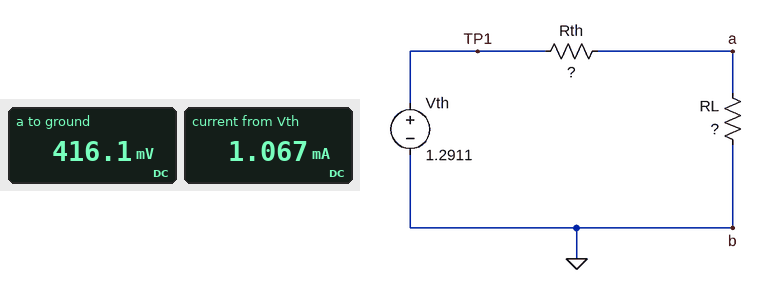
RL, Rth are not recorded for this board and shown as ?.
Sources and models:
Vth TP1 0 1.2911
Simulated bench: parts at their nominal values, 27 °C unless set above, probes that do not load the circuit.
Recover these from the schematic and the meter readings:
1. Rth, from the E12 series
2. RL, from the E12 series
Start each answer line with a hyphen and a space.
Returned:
- 820 Ω
- 390 Ω
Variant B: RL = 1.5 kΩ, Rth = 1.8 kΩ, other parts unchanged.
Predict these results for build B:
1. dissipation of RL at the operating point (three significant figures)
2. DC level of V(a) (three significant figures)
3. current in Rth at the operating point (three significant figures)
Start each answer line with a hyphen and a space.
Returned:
- 230 µW
- 587 mV
- 391 µA
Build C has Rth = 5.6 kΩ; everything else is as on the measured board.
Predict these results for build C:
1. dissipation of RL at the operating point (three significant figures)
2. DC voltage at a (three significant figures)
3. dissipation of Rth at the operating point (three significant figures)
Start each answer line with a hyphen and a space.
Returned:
- 18.1 µW
- 84.1 mV
- 260 µW
